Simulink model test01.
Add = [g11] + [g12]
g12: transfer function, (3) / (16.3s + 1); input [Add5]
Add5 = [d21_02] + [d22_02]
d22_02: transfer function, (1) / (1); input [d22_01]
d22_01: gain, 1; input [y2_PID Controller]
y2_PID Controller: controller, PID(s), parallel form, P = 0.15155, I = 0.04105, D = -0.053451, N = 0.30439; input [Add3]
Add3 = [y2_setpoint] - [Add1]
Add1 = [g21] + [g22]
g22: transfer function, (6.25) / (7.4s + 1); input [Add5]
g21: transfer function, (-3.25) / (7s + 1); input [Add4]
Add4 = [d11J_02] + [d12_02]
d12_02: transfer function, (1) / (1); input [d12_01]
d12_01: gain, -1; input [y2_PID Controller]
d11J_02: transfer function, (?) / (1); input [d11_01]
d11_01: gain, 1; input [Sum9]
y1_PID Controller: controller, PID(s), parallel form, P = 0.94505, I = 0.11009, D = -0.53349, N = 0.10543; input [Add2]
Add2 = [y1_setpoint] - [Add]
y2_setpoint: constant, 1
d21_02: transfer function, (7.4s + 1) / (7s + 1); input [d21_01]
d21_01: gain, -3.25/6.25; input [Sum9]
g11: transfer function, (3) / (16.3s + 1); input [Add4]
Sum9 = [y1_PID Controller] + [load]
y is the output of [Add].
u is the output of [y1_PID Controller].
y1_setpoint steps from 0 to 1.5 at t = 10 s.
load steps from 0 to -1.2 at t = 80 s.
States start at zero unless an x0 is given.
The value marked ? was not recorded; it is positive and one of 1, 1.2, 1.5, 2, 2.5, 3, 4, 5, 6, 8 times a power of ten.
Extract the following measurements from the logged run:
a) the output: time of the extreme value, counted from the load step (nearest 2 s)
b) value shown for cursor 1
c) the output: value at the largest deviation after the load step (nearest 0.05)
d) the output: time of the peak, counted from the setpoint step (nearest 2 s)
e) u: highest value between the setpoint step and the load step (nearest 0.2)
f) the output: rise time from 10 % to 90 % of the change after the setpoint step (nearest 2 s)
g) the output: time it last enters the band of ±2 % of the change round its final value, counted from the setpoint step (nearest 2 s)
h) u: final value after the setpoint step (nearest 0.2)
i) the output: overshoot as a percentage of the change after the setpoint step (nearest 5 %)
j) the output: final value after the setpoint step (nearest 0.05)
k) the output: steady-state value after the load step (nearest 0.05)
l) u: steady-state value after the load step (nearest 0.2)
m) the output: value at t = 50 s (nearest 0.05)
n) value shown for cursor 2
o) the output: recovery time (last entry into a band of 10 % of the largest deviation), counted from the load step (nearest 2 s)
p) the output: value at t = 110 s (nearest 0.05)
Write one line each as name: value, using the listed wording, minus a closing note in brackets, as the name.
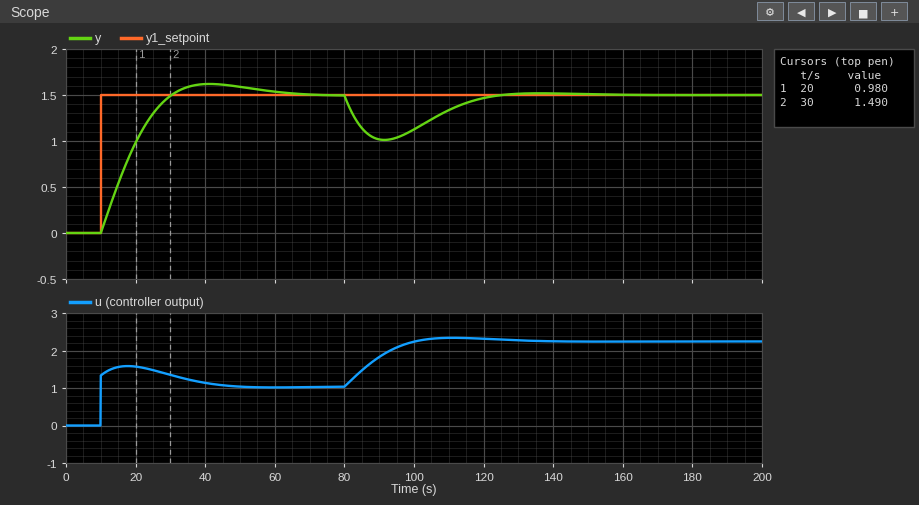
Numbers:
the output: time of the extreme value, counted from the load step: 12 s
value shown for cursor 1: 0.980
the output: value at the largest deviation after the load step: 1.00
the output: time of the peak, counted from the setpoint step: 32 s
u: highest value between the setpoint step and the load step: 1.6
the output: rise time from 10 % to 90 % of the change after the setpoint step: 14 s
the output: time it last enters the band of ±2 % of the change round its final value, counted from the setpoint step: 52 s
u: final value after the setpoint step: 1.0
the output: overshoot as a percentage of the change after the setpoint step: 10 %
the output: final value after the setpoint step: 1.50
the output: steady-state value after the load step: 1.50
u: steady-state value after the load step: 2.2
the output: value at t = 50 s: 1.60
value shown for cursor 2: 1.490
the output: recovery time (last entry into a band of 10 % of the largest deviation), counted from the load step: 38 s
the output: value at t = 110 s: 1.35
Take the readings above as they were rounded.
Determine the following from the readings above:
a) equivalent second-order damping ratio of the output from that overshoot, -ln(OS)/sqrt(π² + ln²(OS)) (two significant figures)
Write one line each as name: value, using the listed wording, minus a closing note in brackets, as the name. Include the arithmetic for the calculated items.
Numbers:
equivalent second-order damping ratio of the output from that overshoot, -ln(OS)/sqrt(π² + ln²(OS)): ln(0.1) = -2.303; 2.303 / sqrt(9.870 + 5.302) = 0.59
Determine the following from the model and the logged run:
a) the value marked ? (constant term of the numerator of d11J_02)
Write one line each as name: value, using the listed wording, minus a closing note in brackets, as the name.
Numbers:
the value marked ?: 1
